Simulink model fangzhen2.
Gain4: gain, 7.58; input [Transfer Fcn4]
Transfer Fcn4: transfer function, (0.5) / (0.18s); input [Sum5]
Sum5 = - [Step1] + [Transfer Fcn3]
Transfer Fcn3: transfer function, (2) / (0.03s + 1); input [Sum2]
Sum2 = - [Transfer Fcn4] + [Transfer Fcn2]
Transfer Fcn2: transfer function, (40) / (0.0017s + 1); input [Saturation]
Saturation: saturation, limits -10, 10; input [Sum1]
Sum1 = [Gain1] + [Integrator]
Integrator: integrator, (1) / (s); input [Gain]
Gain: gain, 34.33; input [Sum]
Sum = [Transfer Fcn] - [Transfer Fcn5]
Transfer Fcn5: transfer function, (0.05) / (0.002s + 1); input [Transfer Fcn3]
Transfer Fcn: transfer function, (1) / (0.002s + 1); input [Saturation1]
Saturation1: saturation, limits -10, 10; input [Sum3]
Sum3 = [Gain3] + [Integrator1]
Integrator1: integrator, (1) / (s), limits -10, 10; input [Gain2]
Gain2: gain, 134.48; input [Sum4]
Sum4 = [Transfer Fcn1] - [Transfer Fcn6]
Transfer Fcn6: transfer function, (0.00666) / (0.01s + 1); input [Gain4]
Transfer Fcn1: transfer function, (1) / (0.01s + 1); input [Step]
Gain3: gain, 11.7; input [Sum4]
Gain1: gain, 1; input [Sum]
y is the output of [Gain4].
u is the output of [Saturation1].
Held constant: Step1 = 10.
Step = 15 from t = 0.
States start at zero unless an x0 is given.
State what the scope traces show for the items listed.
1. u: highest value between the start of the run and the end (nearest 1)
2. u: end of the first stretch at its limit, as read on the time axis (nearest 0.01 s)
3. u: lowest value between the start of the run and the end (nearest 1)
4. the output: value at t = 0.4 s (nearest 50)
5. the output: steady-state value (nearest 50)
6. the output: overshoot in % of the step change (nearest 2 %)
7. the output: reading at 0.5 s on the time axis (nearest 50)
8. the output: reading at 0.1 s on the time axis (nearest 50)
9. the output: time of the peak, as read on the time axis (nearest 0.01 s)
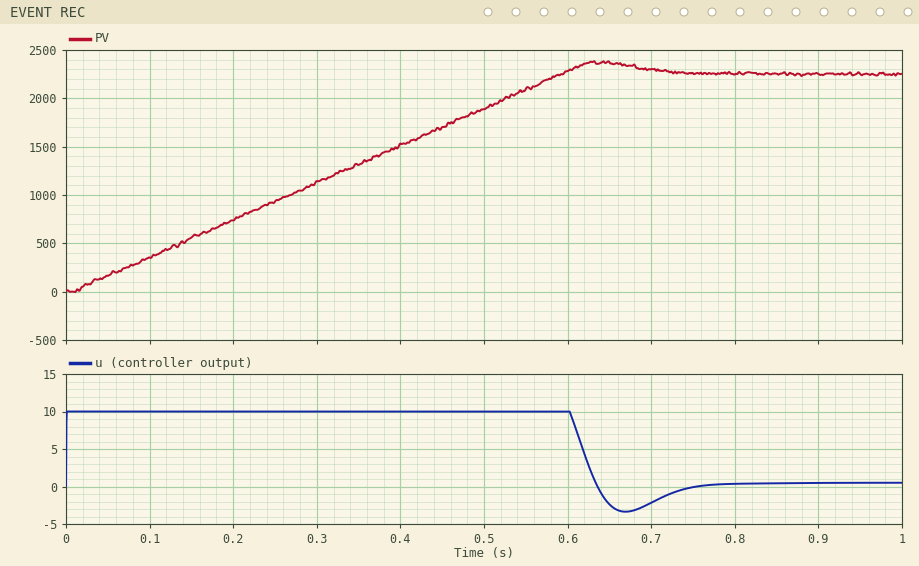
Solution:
10
0.60 s
-3
1500
2250
6 %
1900
350
0.64 s
